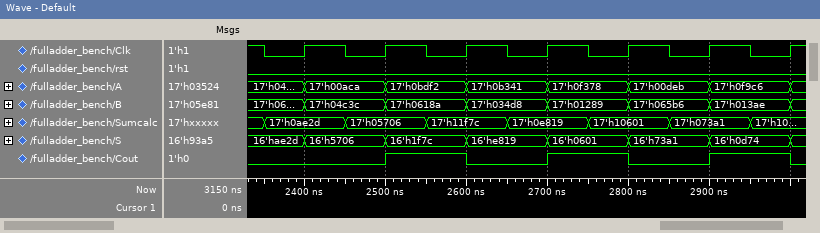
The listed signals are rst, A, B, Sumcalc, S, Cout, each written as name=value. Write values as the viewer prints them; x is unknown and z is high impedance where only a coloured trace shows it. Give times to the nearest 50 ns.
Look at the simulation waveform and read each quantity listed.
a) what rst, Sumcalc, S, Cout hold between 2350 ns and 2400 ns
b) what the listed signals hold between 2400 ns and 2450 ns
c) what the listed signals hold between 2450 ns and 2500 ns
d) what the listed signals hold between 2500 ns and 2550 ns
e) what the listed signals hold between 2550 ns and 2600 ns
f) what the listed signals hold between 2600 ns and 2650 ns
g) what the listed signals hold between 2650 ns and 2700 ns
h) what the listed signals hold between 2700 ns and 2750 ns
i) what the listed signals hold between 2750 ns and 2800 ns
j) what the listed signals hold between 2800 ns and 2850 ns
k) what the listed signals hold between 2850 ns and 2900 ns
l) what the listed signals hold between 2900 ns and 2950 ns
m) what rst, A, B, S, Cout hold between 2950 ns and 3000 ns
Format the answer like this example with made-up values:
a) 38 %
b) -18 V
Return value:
a) rst=0, Sumcalc=17'h0ae2d, S=16'hae2d, Cout=0
b) rst=0, A=17'h00aca, B=17'h04c3c, Sumcalc=17'h0ae2d, S=16'h5706, Cout=0
c) rst=0, A=17'h00aca, B=17'h04c3c, Sumcalc=17'h05706, S=16'h5706, Cout=0
d) rst=0, A=17'h0bdf2, B=17'h0618a, Sumcalc=17'h05706, S=16'h1f7c, Cout=1
e) rst=0, A=17'h0bdf2, B=17'h0618a, Sumcalc=17'h11f7c, S=16'h1f7c, Cout=1
f) rst=0, A=17'h0b341, B=17'h034d8, Sumcalc=17'h11f7c, S=16'he819, Cout=0
g) rst=0, A=17'h0b341, B=17'h034d8, Sumcalc=17'h0e819, S=16'he819, Cout=0
h) rst=0, A=17'h0f378, B=17'h01289, Sumcalc=17'h0e819, S=16'h0601, Cout=1
i) rst=0, A=17'h0f378, B=17'h01289, Sumcalc=17'h10601, S=16'h0601, Cout=1
j) rst=0, A=17'h00deb, B=17'h065b6, Sumcalc=17'h10601, S=16'h73a1, Cout=0
k) rst=0, A=17'h00deb, B=17'h065b6, Sumcalc=17'h073a1, S=16'h73a1, Cout=0
l) rst=0, A=17'h0f9c6, B=17'h013ae, Sumcalc=17'h073a1, S=16'h0d74, Cout=1
m) rst=0, A=17'h0f9c6, B=17'h013ae, S=16'h0d74, Cout=1
